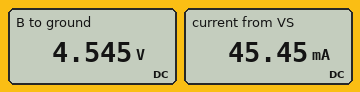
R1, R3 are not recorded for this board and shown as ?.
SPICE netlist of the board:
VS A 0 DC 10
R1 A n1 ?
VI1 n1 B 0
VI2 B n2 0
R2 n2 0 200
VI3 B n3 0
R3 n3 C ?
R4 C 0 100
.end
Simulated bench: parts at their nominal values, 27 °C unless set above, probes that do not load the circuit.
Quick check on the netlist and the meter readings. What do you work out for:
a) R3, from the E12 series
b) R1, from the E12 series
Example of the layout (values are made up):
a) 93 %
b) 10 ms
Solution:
a) 100 Ω
b) 120 Ω
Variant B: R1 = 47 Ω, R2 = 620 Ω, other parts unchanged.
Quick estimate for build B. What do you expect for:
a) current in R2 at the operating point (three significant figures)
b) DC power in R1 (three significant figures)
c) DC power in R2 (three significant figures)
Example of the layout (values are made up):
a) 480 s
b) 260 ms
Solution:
a) 12.3 mA
b) 120 mW
c) 93.9 mW
